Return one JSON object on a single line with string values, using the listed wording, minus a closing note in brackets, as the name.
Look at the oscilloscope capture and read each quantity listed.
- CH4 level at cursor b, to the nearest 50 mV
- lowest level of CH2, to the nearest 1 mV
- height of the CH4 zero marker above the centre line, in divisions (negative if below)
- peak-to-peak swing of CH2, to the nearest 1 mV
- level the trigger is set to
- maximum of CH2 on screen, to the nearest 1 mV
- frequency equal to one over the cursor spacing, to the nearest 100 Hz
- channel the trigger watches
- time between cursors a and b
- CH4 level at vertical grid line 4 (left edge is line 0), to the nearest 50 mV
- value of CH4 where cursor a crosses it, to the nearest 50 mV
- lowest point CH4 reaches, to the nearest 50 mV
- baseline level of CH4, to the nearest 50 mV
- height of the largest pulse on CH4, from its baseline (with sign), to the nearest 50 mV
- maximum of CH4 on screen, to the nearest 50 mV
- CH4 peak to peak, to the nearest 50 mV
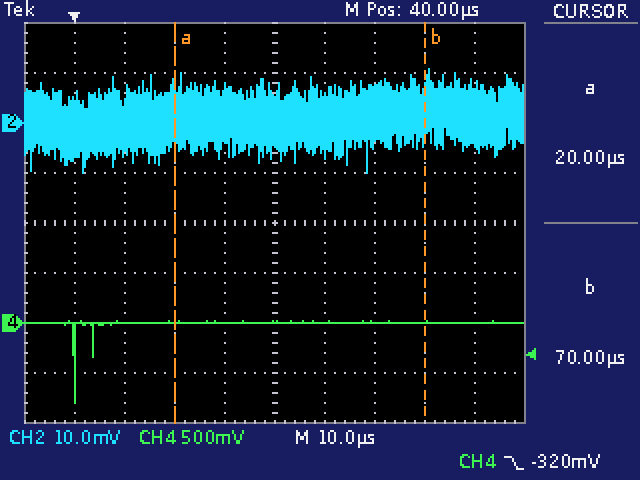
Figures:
{"CH4 level at cursor b, to the nearest 50 mV": "0 mV", "lowest level of CH2, to the nearest 1 mV": "-10 mV", "height of the CH4 zero marker above the centre line, in divisions": "-2.0 div", "peak-to-peak swing of CH2, to the nearest 1 mV": "21 mV", "level the trigger is set to": "-320 mV", "maximum of CH2 on screen, to the nearest 1 mV": "11 mV", "frequency equal to one over the cursor spacing, to the nearest 100 Hz": "20.0 kHz", "channel the trigger watches": "CH4", "time between cursors a and b": "50 µs", "CH4 level at vertical grid line 4 (left edge is line 0), to the nearest 50 mV": "0 mV", "value of CH4 where cursor a crosses it, to the nearest 50 mV": "0 mV", "lowest point CH4 reaches, to the nearest 50 mV": "-800 mV", "baseline level of CH4, to the nearest 50 mV": "0 mV", "height of the largest pulse on CH4, from its baseline (with sign), to the nearest 50 mV": "-800 mV", "maximum of CH4 on screen, to the nearest 50 mV": "0 mV", "CH4 peak to peak, to the nearest 50 mV": "800 mV"}
